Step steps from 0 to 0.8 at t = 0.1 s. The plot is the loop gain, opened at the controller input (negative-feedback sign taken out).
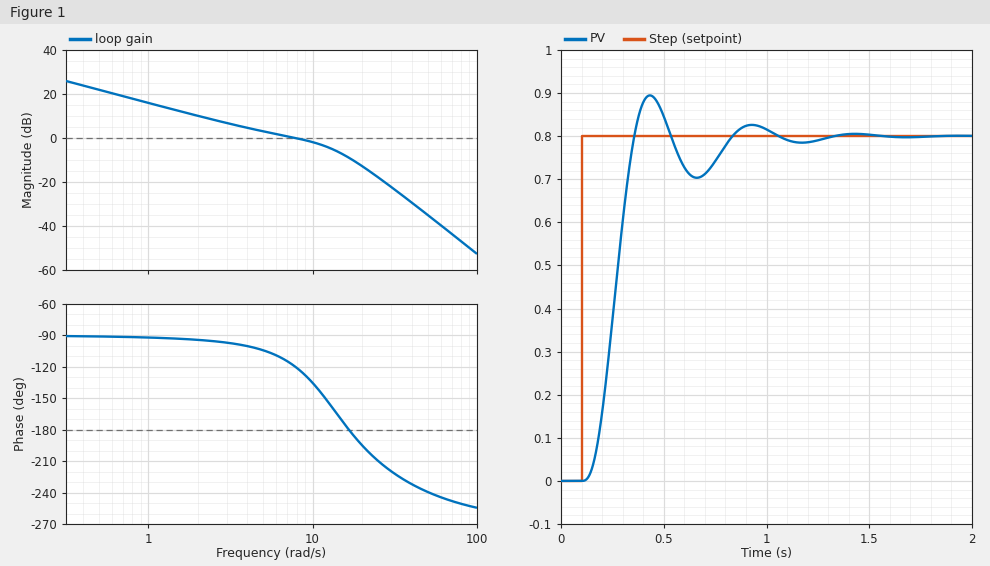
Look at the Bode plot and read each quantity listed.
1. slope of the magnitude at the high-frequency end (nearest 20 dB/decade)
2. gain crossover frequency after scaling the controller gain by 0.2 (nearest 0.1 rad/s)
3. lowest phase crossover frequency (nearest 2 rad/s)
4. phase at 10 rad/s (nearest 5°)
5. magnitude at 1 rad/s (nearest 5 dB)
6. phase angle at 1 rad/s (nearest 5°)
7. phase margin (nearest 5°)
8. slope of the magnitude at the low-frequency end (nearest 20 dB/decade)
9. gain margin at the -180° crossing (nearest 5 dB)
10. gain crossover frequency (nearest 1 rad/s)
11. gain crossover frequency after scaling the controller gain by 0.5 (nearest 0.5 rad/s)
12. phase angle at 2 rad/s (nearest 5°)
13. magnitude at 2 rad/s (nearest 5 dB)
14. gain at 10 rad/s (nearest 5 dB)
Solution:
-60 dB/decade
1.3 rad/s
16 rad/s
-135°
15 dB
-90°
60°
-20 dB/decade
10 dB
8 rad/s
3.5 rad/s
-95°
10 dB
0 dB
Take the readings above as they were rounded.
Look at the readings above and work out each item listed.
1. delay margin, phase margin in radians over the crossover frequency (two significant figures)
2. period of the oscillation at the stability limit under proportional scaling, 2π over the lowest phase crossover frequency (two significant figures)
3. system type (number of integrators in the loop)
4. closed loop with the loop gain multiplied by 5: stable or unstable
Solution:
0.13 s
0.39 s
1
unstable
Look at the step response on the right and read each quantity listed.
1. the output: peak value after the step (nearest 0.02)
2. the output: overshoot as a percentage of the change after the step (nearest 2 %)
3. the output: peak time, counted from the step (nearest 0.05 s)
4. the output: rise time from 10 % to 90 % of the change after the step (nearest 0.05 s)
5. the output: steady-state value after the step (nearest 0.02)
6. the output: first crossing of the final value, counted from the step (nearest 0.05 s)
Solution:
0.90
12 %
0.35 s
0.15 s
0.80
0.25 s
